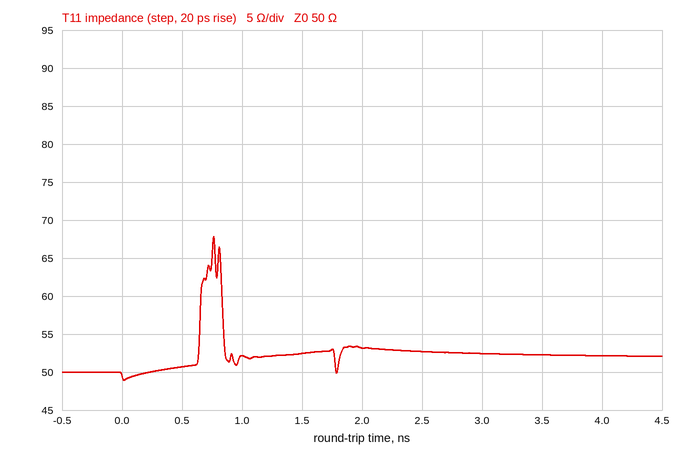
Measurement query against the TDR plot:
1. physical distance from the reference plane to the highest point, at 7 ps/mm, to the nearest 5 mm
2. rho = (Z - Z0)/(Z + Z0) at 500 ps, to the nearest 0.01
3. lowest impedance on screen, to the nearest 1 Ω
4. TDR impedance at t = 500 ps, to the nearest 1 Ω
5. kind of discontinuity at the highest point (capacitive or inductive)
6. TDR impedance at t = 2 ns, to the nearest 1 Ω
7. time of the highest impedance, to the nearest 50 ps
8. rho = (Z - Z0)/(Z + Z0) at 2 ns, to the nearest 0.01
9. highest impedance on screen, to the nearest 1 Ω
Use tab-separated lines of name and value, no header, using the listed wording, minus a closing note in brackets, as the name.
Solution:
physical distance from the reference plane to the highest point, at 7 ps/mm, to the nearest 5 mm	55 mm
rho = (Z - Z0)/(Z + Z0) at 500 ps, to the nearest 0.01	+0.01
lowest impedance on screen, to the nearest 1 Ω	49 Ω
TDR impedance at t = 500 ps, to the nearest 1 Ω	51 Ω
kind of discontinuity at the highest point	inductive
TDR impedance at t = 2 ns, to the nearest 1 Ω	53 Ω
time of the highest impedance, to the nearest 50 ps	750 ps
rho = (Z - Z0)/(Z + Z0) at 2 ns, to the nearest 0.01	+0.03
highest impedance on screen, to the nearest 1 Ω	68 Ω
